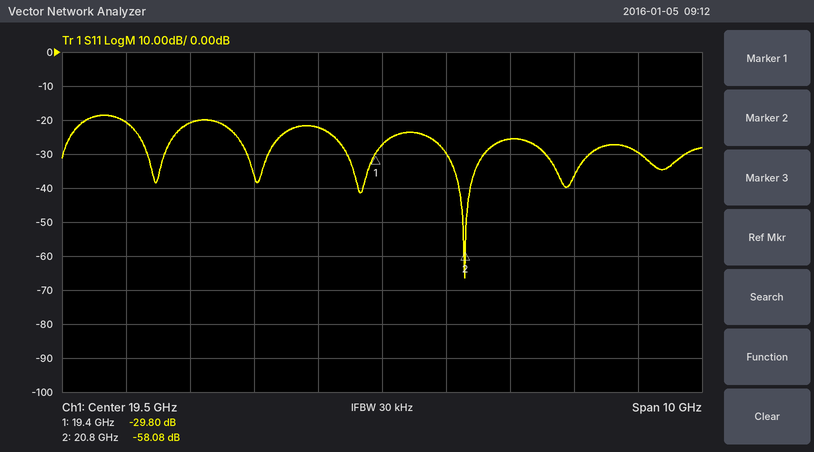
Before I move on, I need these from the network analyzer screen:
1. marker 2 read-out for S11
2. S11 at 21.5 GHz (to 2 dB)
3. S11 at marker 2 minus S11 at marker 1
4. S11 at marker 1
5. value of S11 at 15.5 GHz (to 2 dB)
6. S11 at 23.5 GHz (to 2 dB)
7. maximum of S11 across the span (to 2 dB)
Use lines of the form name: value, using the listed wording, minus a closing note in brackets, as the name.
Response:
marker 2 read-out for S11: -58.08 dB
S11 at 21.5 GHz: -26 dB
S11 at marker 2 minus S11 at marker 1: -28.28 dB
S11 at marker 1: -29.80 dB
value of S11 at 15.5 GHz: -20 dB
S11 at 23.5 GHz: -30 dB
maximum of S11 across the span: -18 dB
